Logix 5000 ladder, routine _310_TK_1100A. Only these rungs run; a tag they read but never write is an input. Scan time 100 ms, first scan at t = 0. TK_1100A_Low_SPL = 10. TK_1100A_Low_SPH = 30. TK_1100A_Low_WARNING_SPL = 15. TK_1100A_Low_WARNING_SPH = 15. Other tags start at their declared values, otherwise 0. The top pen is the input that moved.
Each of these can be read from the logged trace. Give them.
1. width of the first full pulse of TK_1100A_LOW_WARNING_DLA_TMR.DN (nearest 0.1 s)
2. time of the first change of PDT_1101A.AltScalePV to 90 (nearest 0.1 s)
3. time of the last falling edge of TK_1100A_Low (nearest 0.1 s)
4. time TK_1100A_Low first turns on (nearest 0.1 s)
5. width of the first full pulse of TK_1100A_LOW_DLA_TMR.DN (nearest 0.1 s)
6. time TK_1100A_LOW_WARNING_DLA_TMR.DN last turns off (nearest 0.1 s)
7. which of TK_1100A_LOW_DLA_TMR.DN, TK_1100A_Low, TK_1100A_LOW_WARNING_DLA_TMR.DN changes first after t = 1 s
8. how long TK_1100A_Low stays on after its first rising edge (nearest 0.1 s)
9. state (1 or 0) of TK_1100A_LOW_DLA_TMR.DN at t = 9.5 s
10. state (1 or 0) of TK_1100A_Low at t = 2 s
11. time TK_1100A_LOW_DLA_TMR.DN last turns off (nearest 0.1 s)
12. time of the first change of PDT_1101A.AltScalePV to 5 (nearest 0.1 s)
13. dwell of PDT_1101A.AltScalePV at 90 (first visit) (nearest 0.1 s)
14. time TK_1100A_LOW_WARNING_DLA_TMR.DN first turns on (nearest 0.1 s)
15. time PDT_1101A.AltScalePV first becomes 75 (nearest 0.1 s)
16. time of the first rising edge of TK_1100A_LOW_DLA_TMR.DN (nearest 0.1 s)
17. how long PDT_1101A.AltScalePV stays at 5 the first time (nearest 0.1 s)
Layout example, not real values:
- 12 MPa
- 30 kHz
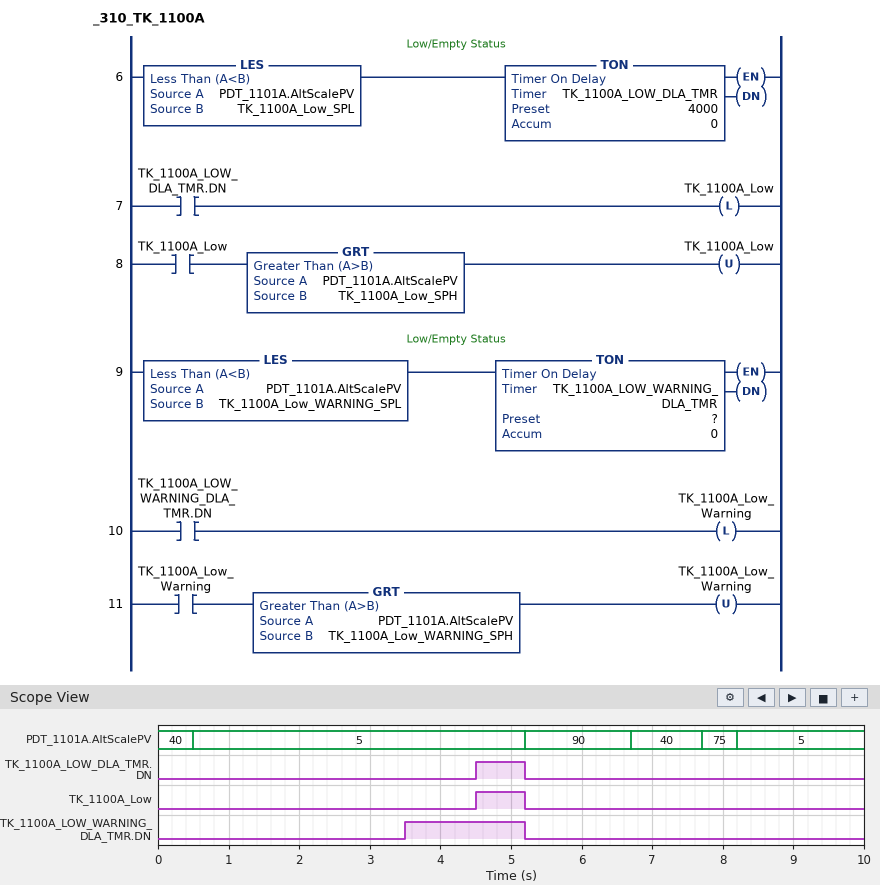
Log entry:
- 1.7 s
- 5.2 s
- 5.2 s
- 4.5 s
- 0.7 s
- 5.2 s
- TK_1100A_LOW_WARNING_DLA_TMR.DN
- 0.7 s
- 0
- 0
- 5.2 s
- 0.5 s
- 1.5 s
- 3.5 s
- 7.7 s
- 4.5 s
- 4.7 s
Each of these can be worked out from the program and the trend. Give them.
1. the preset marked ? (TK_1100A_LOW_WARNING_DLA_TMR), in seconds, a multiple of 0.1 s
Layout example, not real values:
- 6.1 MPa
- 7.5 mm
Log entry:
- 3.0 s
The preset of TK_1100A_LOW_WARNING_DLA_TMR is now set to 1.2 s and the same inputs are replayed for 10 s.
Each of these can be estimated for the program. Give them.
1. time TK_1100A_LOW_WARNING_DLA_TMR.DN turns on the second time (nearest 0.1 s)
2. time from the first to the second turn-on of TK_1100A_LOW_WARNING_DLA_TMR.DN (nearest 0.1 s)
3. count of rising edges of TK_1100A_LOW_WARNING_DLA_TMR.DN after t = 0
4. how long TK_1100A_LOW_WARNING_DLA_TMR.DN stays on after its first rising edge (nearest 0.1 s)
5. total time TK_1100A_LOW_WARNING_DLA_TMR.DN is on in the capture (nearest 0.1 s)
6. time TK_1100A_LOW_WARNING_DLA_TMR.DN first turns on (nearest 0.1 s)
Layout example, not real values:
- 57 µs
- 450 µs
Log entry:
- 9.4 s
- 7.7 s
- 2
- 3.5 s
- 4.1 s
- 1.7 s
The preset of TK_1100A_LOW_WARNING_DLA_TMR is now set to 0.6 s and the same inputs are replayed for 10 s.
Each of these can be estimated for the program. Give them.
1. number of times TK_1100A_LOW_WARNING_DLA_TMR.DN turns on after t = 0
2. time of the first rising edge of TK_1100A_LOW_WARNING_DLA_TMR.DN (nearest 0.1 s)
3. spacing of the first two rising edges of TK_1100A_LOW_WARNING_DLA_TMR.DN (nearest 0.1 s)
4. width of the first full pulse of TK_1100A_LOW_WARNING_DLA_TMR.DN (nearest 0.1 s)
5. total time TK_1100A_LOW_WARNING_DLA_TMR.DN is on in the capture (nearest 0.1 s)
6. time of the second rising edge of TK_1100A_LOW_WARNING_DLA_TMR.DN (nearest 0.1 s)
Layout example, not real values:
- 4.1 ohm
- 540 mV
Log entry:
- 2
- 1.1 s
- 7.7 s
- 4.1 s
- 5.3 s
- 8.8 s
